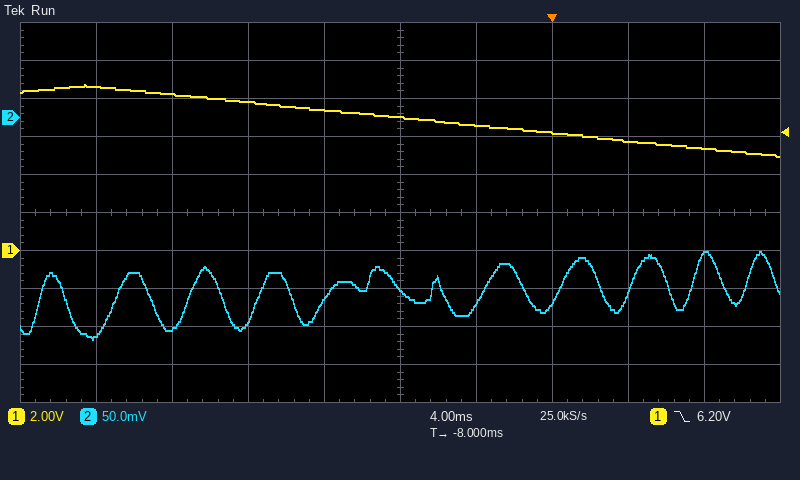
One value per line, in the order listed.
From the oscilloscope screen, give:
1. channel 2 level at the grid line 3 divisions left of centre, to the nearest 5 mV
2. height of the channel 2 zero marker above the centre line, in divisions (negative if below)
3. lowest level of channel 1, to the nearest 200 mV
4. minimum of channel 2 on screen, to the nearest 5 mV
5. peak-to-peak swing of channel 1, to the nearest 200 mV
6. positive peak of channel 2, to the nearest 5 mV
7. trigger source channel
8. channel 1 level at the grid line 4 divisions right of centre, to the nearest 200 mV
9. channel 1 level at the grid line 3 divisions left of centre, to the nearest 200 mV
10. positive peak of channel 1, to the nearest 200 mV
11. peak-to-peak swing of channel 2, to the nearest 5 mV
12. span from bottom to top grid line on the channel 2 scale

-280 mV
+2.5 div
5.0 V
-290 mV
3.8 V
-175 mV
channel 1
5.4 V
8.2 V
8.8 V
115 mV
500 mV
